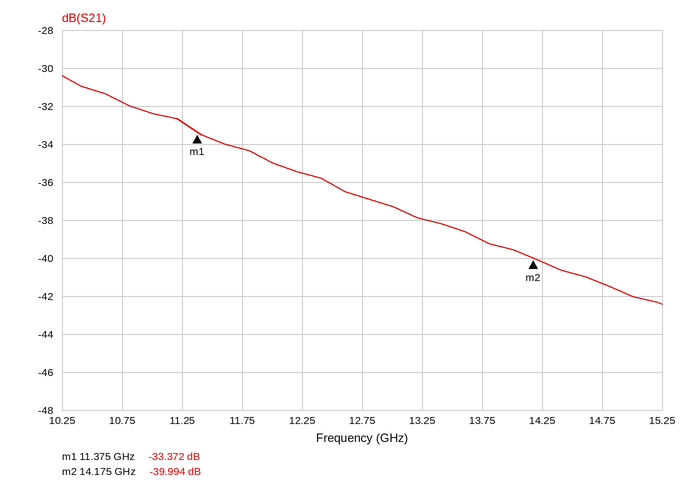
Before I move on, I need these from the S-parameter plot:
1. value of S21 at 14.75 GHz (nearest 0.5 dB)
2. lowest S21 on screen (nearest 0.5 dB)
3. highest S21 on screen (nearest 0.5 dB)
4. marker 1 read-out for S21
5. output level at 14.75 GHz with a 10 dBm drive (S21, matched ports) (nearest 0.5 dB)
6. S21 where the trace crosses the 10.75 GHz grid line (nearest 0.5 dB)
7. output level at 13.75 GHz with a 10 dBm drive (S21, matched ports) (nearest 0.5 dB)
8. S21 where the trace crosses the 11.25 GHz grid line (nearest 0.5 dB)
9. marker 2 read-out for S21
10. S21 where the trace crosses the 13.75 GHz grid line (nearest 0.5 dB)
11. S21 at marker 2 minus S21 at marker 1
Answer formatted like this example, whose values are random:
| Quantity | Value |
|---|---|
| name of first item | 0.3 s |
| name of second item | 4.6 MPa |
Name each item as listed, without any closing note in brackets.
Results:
| Quantity | Value |
|---|---|
| value of S21 at 14.75 GHz | -41.5 dB |
| lowest S21 on screen | -42.5 dB |
| highest S21 on screen | -30.5 dB |
| marker 1 read-out for S21 | -33.372 dB |
| output level at 14.75 GHz with a 10 dBm drive (S21, matched ports) | -31.5 dBm |
| S21 where the trace crosses the 10.75 GHz grid line | -32.0 dB |
| output level at 13.75 GHz with a 10 dBm drive (S21, matched ports) | -29.0 dBm |
| S21 where the trace crosses the 11.25 GHz grid line | -33.0 dB |
| marker 2 read-out for S21 | -39.994 dB |
| S21 where the trace crosses the 13.75 GHz grid line | -39.0 dB |
| S21 at marker 2 minus S21 at marker 1 | -6.622 dB |
